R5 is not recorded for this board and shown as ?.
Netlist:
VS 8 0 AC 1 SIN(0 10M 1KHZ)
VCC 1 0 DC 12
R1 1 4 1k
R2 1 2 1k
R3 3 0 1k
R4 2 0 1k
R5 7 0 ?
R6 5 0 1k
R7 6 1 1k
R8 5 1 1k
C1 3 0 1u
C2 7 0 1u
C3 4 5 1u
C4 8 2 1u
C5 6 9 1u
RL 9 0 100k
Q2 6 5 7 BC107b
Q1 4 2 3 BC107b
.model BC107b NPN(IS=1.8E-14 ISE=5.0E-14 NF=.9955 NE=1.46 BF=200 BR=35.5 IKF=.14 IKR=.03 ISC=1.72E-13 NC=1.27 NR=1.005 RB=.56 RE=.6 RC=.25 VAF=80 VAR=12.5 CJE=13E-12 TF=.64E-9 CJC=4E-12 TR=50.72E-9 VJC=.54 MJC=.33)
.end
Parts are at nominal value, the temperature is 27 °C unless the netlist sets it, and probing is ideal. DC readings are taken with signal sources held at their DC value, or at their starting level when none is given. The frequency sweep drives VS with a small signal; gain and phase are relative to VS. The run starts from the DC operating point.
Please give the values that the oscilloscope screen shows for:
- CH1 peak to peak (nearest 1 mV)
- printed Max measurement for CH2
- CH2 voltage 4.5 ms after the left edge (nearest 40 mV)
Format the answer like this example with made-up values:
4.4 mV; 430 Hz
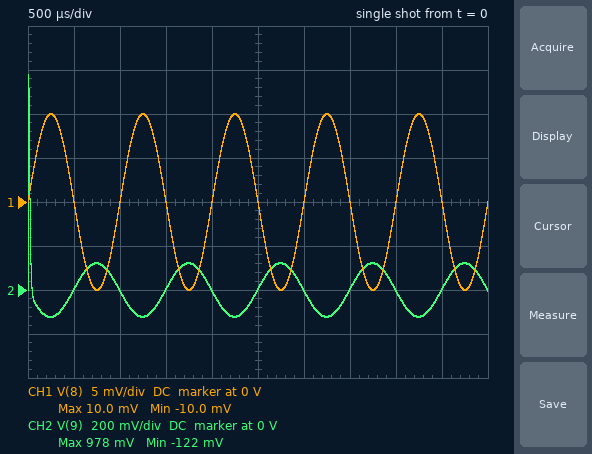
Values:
20 mV; 978 mV; 0 V
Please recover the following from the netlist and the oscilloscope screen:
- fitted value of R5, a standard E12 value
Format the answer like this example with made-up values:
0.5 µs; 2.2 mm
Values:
1.2 kΩ
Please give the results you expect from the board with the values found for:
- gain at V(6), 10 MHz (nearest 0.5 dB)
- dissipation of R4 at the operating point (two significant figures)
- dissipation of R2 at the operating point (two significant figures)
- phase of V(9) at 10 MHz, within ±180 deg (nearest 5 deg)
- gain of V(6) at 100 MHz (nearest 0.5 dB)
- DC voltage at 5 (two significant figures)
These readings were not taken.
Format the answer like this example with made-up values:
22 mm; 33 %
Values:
58.0 dB; 36 mW; 36 mW; -85 deg; 37.5 dB; 6.0 V
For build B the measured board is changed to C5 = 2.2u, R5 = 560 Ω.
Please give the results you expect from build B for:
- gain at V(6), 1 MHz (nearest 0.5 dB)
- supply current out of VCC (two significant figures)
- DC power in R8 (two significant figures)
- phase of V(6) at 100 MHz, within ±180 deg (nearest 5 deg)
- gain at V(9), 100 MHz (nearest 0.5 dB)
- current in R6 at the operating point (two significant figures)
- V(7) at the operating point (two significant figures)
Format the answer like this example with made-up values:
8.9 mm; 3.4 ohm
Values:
-8.0 dB; 25 mA; 43 mW; 160 deg; -9.5 dB; 5.4 mA; 4.7 V
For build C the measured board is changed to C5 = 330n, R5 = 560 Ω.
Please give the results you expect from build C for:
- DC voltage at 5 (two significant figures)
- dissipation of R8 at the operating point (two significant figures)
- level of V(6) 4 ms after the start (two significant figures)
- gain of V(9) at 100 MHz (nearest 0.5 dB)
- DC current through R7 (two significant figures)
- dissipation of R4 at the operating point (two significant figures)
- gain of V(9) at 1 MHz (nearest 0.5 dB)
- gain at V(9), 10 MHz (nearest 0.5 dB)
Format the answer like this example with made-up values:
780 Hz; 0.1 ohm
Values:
5.4 V; 43 mW; 4.7 V; -9.5 dB; 7.3 mA; 36 mW; -8.0 dB; -9.0 dB
